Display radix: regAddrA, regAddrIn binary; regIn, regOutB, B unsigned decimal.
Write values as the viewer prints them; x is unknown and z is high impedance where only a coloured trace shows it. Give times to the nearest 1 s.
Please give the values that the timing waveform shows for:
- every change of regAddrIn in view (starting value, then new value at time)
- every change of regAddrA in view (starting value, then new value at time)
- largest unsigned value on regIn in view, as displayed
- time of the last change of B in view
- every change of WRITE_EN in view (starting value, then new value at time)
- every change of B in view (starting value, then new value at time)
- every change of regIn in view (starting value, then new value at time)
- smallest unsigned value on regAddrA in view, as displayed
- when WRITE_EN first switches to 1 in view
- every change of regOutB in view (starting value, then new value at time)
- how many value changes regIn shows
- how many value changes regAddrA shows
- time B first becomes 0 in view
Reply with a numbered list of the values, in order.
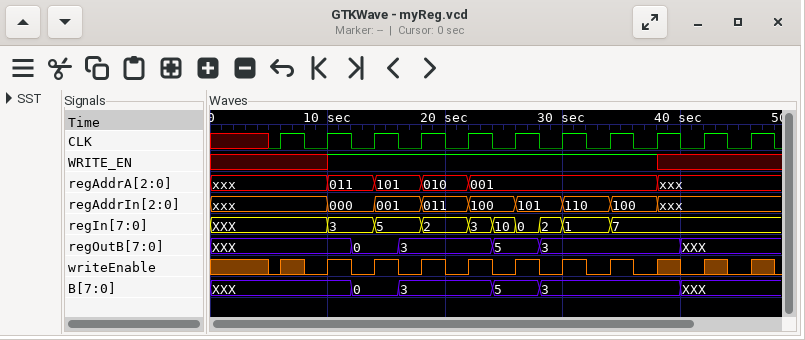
1. xxx, 000 at 10 s, 001 at 14 s, 011 at 18 s, 100 at 22 s, 101 at 26 s, 110 at 30 s, 100 at 34 s, xxx at 38 s
2. xxx, 011 at 10 s, 101 at 14 s, 010 at 18 s, 001 at 22 s, xxx at 38 s
3. 10
4. 40 s
5. x, 1 at 10 s, x at 38 s
6. XXX, 0 at 12 s, 3 at 16 s, 5 at 24 s, 3 at 28 s, XXX at 40 s
7. XXX, 3 at 10 s, 5 at 14 s, 2 at 18 s, 3 at 22 s, 10 at 24 s, 0 at 26 s, 2 at 28 s, 1 at 30 s, 7 at 34 s
8. 001
9. 10 s
10. XXX, 0 at 12 s, 3 at 16 s, 5 at 24 s, 3 at 28 s, XXX at 40 s
11. 9
12. 5
13. 12 s
